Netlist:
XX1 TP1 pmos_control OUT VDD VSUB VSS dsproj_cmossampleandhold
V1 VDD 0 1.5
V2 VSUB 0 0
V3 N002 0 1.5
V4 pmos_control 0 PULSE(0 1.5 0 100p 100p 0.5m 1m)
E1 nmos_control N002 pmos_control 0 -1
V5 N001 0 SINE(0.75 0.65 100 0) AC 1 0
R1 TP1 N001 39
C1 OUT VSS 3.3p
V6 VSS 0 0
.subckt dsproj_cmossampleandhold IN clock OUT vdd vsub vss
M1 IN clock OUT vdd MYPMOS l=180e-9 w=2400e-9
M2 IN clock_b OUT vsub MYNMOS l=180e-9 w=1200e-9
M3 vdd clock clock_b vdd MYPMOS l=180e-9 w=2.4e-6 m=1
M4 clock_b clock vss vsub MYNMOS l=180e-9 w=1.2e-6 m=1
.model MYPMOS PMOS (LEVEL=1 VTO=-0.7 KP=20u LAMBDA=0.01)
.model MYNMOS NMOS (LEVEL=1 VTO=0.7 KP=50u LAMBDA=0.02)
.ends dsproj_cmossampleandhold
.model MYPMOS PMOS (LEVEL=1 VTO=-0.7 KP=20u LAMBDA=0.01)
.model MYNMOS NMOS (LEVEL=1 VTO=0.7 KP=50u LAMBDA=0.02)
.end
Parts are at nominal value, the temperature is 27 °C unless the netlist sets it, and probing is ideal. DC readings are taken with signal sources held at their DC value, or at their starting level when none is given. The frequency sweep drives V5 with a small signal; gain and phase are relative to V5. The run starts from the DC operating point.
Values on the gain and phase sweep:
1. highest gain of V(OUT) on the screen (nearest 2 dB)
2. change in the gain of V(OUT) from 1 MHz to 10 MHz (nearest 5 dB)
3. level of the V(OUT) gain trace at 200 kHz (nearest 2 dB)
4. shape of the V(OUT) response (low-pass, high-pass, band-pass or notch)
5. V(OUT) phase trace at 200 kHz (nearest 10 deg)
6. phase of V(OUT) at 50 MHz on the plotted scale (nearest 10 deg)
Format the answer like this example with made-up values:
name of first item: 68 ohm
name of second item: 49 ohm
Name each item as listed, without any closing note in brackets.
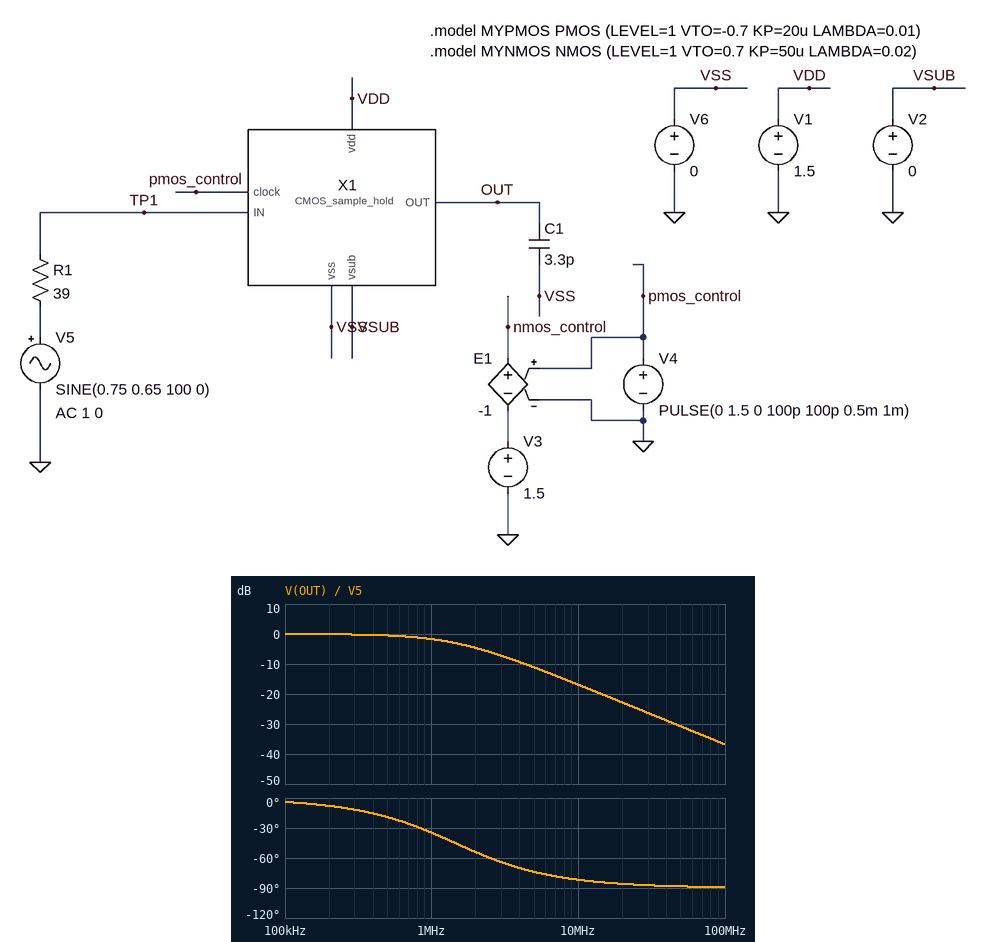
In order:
highest gain of V(OUT) on the screen: 0 dB
change in the gain of V(OUT) from 1 MHz to 10 MHz: -15 dB
level of the V(OUT) gain trace at 200 kHz: 0 dB
shape of the V(OUT) response: low-pass
V(OUT) phase trace at 200 kHz: -10 deg
phase of V(OUT) at 50 MHz on the plotted scale: -90 deg
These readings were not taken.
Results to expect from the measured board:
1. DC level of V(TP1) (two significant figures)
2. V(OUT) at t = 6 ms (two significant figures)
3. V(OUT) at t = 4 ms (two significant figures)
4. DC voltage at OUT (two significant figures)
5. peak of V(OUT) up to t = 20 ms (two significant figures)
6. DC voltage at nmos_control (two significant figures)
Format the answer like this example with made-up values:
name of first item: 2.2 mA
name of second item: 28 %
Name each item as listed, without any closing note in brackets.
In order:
DC level of V(TP1): 750 mV
V(OUT) at t = 6 ms: 370 mV
V(OUT) at t = 4 ms: 1.1 V
DC voltage at OUT: 750 mV
peak of V(OUT) up to t = 20 ms: 1.4 V
DC voltage at nmos_control: 1.5 V
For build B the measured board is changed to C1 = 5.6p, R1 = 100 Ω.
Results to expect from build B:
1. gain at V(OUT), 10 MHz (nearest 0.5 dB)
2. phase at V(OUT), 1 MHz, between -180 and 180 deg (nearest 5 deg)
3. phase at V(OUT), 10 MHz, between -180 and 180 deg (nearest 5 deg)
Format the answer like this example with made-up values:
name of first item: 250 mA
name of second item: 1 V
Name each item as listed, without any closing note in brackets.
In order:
gain at V(OUT), 10 MHz: -21.5 dB
phase at V(OUT), 1 MHz, between -180 and 180 deg: -50 deg
phase at V(OUT), 10 MHz, between -180 and 180 deg: -85 deg
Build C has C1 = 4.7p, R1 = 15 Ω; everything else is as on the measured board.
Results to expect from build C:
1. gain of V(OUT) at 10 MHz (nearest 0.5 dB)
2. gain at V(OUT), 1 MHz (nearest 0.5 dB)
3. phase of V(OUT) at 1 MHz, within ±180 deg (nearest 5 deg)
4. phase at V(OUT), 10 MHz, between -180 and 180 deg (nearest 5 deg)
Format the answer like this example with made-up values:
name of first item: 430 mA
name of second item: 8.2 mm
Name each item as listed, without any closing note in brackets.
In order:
gain of V(OUT) at 10 MHz: -20.0 dB
gain at V(OUT), 1 MHz: -3.0 dB
phase of V(OUT) at 1 MHz, within ±180 deg: -45 deg
phase at V(OUT), 10 MHz, between -180 and 180 deg: -85 deg
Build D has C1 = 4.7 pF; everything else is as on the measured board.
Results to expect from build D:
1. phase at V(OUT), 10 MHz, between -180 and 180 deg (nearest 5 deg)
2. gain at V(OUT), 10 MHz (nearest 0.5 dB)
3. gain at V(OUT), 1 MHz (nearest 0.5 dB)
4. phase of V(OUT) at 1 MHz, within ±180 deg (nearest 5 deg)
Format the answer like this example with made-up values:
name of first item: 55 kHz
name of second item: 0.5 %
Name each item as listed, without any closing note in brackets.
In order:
phase at V(OUT), 10 MHz, between -180 and 180 deg: -85 deg
gain at V(OUT), 10 MHz: -20.0 dB
gain at V(OUT), 1 MHz: -3.0 dB
phase of V(OUT) at 1 MHz, within ±180 deg: -45 deg
